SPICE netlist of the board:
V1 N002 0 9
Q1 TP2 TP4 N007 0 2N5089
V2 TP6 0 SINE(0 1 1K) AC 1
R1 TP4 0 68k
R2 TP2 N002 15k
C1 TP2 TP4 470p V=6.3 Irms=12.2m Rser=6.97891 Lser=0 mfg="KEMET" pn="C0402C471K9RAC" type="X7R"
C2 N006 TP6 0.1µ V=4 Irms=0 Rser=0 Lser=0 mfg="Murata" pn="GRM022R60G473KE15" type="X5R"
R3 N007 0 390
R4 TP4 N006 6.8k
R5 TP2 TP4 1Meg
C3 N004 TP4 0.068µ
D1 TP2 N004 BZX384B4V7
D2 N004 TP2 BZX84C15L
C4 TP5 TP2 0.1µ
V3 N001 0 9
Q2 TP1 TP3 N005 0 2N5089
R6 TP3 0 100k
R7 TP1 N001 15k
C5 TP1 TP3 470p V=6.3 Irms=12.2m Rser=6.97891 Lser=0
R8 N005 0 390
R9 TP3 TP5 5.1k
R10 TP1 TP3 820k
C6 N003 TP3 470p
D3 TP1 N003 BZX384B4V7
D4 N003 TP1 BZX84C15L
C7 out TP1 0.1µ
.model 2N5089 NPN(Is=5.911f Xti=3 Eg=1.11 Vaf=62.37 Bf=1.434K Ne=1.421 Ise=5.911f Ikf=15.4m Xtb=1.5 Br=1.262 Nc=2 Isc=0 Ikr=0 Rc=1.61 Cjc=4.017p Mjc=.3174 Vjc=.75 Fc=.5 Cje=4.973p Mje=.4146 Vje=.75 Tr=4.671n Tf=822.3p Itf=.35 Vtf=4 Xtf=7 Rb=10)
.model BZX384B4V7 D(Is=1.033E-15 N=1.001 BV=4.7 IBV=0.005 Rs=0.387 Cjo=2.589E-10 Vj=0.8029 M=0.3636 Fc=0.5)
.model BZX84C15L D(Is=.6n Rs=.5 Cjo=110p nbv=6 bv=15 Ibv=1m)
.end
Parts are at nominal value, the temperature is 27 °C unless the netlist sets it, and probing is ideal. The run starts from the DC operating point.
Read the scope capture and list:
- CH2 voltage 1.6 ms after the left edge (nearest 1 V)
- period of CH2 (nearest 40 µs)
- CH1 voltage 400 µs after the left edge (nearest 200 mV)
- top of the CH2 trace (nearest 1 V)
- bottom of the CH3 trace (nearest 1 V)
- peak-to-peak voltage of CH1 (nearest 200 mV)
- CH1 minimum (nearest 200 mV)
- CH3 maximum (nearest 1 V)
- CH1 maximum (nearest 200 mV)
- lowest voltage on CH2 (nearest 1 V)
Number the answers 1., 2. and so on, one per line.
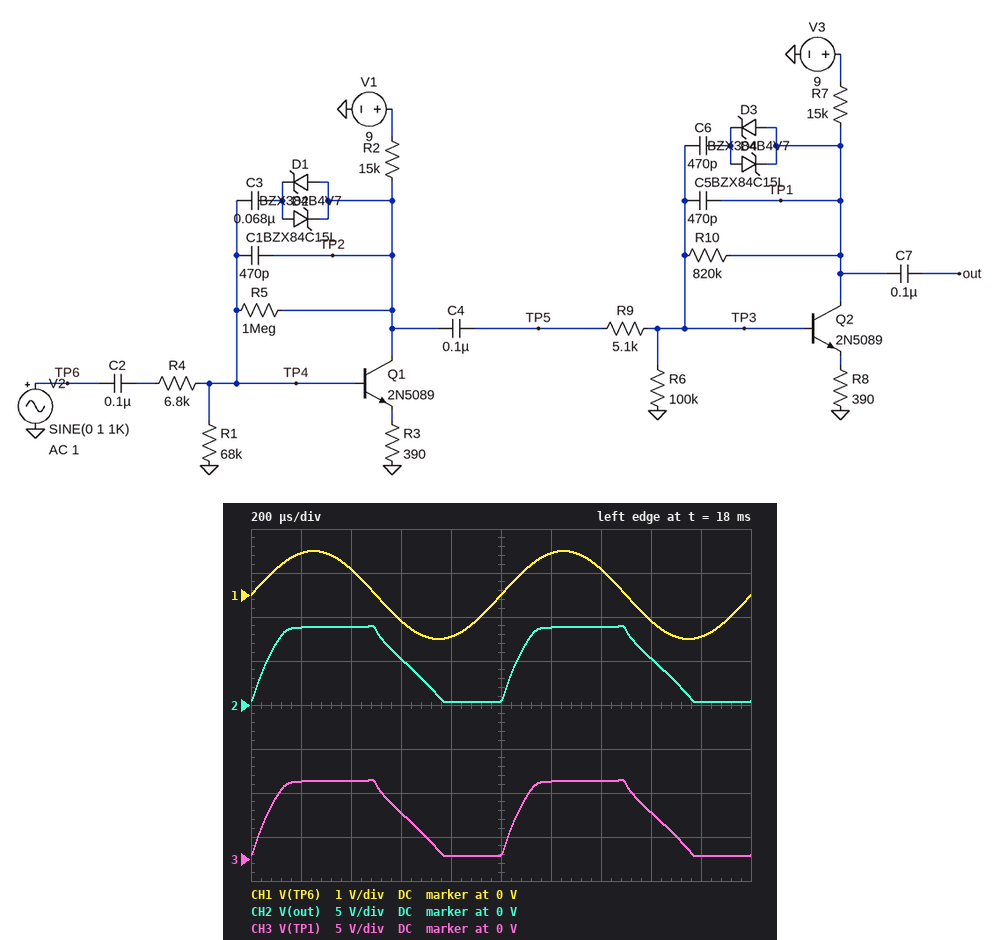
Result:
1. 5 V
2. 1.00 ms
3. 600 mV
4. 9 V
5. 0 V
6. 2.0 V
7. -1.0 V
8. 9 V
9. 1.0 V
10. 0 V
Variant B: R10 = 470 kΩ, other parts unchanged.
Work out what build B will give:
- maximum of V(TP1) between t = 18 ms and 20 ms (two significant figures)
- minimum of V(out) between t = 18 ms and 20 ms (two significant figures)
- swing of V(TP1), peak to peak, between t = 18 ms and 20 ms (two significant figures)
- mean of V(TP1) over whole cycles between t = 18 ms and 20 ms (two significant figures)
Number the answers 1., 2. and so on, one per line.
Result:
1. 8.9 V
2. 310 mV
3. 8.6 V
4. 4.7 V
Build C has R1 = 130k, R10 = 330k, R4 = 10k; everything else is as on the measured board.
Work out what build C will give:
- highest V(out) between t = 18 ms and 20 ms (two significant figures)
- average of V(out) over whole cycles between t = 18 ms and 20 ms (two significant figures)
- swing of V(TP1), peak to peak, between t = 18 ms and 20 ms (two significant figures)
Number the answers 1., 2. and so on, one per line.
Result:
1. 8.7 V
2. 4.6 V
3. 8.4 V
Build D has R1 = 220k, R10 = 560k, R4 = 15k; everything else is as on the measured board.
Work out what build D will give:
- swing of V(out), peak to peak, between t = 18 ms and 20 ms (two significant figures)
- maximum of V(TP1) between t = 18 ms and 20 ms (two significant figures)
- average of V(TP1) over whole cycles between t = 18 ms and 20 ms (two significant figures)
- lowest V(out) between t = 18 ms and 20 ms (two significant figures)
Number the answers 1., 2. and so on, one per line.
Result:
1. 8.6 V
2. 8.9 V
3. 5.0 V
4. 320 mV
